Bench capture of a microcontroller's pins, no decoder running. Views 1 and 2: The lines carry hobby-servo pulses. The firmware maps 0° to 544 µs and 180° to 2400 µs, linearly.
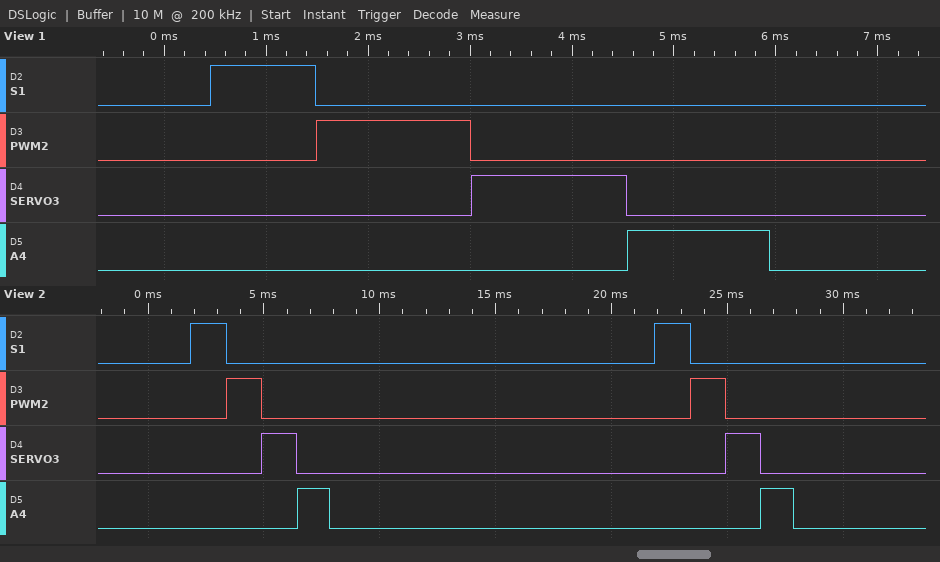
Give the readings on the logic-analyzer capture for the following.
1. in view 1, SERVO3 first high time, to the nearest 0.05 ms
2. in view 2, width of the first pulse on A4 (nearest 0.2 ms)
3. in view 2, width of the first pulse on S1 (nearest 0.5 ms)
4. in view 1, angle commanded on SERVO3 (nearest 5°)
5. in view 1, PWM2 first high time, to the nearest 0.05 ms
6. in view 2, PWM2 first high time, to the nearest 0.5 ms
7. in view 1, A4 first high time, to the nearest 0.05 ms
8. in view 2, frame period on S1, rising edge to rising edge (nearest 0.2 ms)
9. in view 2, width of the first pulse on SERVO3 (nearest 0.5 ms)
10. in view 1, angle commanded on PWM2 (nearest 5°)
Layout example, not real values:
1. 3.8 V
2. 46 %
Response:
1. 1.50 ms
2. 1.4 ms
3. 1.5 ms
4. 95°
5. 1.50 ms
6. 1.5 ms
7. 1.40 ms
8. 20.0 ms
9. 1.5 ms
10. 95°
